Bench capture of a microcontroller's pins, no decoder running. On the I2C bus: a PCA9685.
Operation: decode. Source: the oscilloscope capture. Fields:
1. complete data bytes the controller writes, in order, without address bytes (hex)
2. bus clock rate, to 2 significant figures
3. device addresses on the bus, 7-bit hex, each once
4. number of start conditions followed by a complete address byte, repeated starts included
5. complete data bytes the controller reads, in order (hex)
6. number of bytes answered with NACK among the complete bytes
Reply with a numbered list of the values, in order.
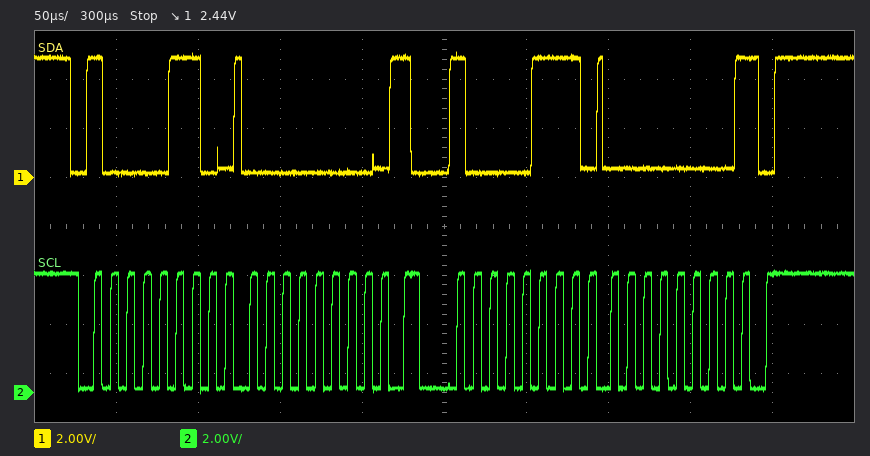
1. 00
2. 100 kHz
3. 0x43
4. 2
5. 00
6. 1
